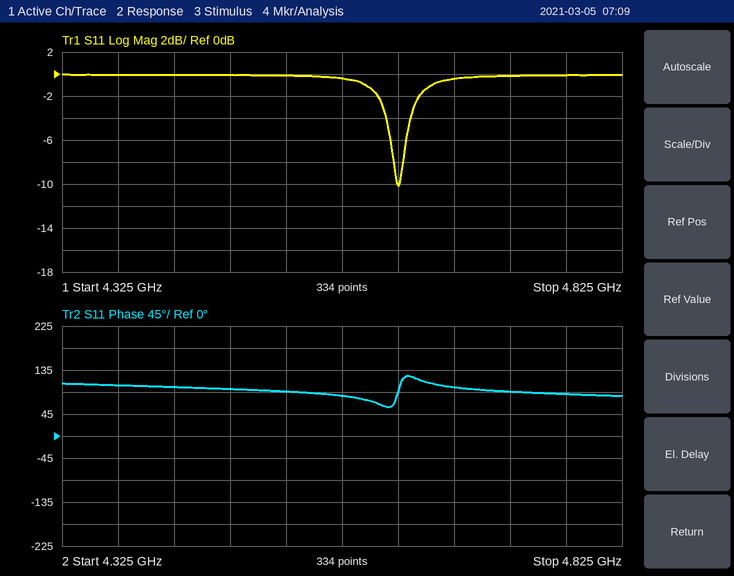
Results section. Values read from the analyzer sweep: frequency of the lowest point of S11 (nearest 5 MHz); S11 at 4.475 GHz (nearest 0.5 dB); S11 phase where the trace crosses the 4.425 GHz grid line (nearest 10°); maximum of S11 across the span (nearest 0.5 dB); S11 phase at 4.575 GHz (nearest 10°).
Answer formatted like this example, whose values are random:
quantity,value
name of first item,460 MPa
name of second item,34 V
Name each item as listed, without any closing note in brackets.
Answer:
quantity,value
frequency of the lowest point of S11,4.625 GHz
S11 at 4.475 GHz,0.0 dB
S11 phase where the trace crosses the 4.425 GHz grid line,100°
maximum of S11 across the span,0.0 dB
S11 phase at 4.575 GHz,80°
